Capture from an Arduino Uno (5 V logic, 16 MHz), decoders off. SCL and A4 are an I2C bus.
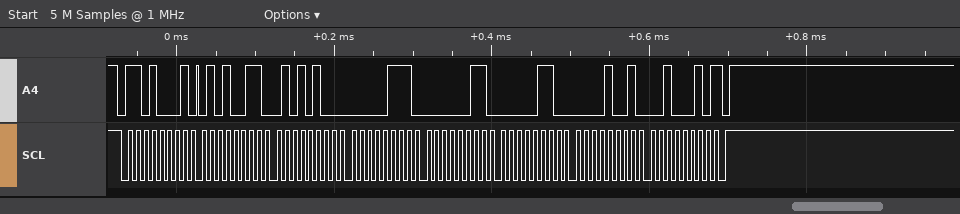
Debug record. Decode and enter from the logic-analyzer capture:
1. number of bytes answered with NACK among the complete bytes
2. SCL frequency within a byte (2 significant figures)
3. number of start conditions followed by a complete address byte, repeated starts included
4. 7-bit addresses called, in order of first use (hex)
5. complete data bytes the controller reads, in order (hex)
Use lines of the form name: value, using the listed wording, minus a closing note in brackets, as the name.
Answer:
number of bytes answered with NACK among the complete bytes: 1
SCL frequency within a byte: 100 kHz
number of start conditions followed by a complete address byte, repeated starts included: 1
7-bit addresses called, in order of first use: 0x68
complete data bytes the controller reads, in order: 53 54 07 03 06 09 22
